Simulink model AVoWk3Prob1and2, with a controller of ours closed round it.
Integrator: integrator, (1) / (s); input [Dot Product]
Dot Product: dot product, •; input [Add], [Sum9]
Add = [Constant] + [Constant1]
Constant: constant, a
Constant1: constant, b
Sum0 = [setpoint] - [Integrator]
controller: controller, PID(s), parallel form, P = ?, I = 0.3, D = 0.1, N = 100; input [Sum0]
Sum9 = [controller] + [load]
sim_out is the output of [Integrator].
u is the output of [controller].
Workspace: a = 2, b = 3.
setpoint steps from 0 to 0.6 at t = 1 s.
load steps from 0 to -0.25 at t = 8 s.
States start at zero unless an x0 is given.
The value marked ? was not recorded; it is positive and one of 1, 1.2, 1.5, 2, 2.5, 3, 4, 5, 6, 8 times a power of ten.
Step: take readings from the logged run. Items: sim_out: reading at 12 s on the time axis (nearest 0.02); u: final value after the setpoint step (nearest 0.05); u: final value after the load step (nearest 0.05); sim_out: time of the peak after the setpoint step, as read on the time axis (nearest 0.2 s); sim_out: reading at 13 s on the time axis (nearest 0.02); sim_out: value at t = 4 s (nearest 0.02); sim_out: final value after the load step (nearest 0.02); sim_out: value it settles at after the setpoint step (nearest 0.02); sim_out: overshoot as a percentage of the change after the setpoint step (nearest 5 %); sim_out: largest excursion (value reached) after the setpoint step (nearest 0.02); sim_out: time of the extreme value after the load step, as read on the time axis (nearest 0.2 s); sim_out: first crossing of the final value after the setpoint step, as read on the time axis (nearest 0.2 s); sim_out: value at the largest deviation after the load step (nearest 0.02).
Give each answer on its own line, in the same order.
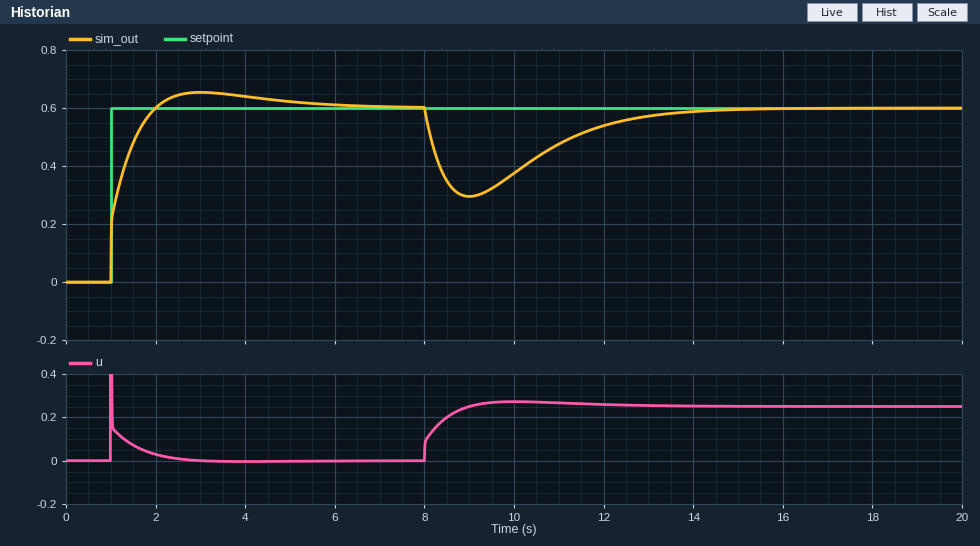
0.54
0.00
0.25
3.0 s
0.58
0.64
0.60
0.60
10 %
0.66
9.0 s
2.0 s
0.30
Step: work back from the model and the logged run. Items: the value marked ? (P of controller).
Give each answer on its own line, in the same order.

0.6
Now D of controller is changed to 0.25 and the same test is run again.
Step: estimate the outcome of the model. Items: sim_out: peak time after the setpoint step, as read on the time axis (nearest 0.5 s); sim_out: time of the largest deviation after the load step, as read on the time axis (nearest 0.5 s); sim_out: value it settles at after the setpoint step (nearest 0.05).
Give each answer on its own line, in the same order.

3.5 s
9.5 s
0.60
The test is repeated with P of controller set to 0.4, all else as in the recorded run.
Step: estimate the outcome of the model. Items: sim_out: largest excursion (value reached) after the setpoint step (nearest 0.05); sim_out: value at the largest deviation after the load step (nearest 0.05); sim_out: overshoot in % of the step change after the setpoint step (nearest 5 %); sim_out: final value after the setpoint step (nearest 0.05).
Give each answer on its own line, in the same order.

0.70
0.20
15 %
0.60
